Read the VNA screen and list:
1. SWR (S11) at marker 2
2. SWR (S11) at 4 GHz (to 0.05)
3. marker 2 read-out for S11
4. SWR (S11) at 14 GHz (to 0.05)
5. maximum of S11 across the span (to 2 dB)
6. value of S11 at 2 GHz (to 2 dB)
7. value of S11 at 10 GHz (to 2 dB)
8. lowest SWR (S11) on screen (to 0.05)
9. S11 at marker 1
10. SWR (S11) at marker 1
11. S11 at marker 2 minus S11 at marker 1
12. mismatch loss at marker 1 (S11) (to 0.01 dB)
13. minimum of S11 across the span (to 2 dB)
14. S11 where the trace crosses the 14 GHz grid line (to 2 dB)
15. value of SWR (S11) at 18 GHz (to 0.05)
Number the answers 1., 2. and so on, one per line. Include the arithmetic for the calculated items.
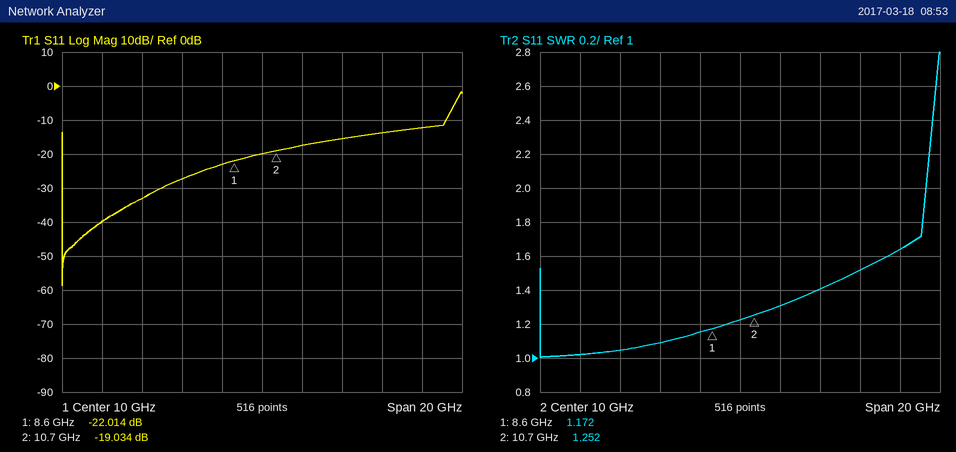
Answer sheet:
1. 1.252
2. 1.05
3. -19.034 dB
4. 1.40
5. -2 dB
6. -40 dB
7. -20 dB
8. 1.00
9. -22.014 dB
10. 1.172
11. -19.034 − (-22.014) = 2.980 dB
12. −10 log10(1 − 10^(-22.014/10)) ≈ 0.03 dB
13. -58 dB
14. -16 dB
15. 1.65
